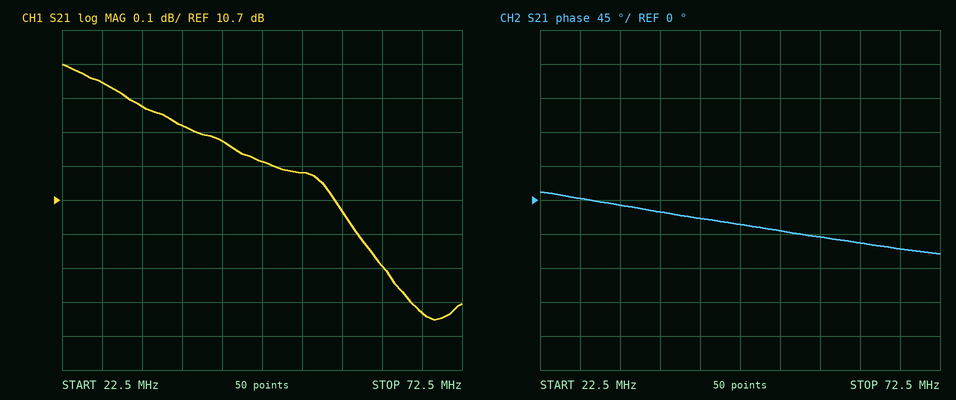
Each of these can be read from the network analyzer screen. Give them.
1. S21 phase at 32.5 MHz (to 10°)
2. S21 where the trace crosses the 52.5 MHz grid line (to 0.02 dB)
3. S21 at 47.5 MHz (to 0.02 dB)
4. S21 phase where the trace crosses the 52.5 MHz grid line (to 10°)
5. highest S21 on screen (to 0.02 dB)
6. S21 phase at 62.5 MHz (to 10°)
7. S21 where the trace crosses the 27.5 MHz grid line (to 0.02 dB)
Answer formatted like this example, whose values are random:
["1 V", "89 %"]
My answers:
["-10°", "10.78 dB", "10.82 dB", "-40°", "11.10 dB", "-60°", "11.04 dB"]
